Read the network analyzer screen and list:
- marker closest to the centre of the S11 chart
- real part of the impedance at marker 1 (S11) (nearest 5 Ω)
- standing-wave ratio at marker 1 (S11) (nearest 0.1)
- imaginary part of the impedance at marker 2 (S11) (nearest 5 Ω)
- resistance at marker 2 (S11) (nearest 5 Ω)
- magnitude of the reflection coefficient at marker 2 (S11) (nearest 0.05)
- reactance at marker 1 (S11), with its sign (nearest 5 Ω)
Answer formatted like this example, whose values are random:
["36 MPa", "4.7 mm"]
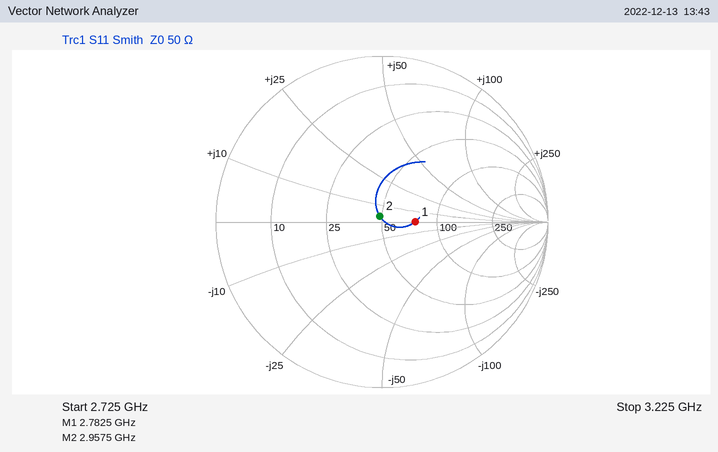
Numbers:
["marker 2", "75 Ω", "1.5", "+5 Ω", "50 Ω", "0.05", "0 Ω"]
